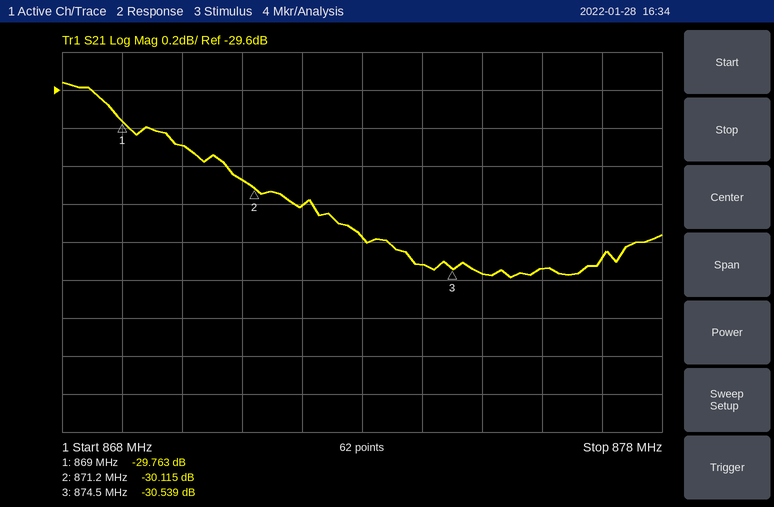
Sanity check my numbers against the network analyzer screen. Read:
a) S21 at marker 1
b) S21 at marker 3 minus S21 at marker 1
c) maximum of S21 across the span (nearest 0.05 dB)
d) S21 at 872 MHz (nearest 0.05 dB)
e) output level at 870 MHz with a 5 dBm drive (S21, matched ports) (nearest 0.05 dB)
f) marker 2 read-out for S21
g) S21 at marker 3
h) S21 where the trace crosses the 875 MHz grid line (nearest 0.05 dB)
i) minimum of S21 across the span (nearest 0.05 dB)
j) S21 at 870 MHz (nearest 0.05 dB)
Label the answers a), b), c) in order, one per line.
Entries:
a) -29.763 dB
b) -0.776 dB
c) -29.55 dB
d) -30.20 dB
e) -24.90 dBm
f) -30.115 dB
g) -30.539 dB
h) -30.55 dB
i) -30.60 dB
j) -29.90 dB
